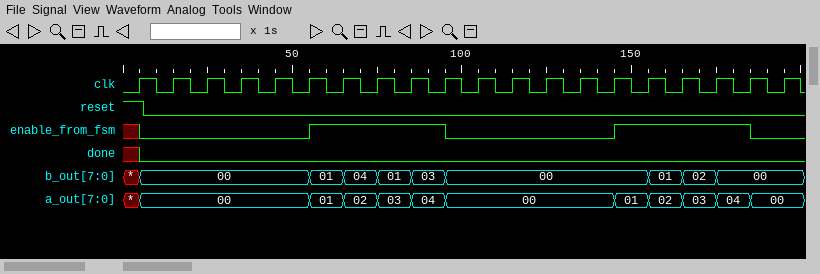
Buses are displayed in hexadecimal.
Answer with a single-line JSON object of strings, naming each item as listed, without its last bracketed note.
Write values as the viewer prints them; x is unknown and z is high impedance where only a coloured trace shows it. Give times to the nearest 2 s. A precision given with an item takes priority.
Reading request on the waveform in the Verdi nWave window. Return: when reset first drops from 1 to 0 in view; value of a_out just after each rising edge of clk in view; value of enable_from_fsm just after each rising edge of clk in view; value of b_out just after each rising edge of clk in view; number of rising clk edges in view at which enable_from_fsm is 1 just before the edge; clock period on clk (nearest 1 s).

{"when reset first drops from 1 to 0 in view": "6 s", "value of a_out just after each rising edge of clk in view": "00, 00, 00, 00, 00, 01, 02, 03, 04, 00, 00, 00, 00, 00, 01, 02, 03, 04, 00, 00", "value of enable_from_fsm just after each rising edge of clk in view": "0 0 0 0 0 1 1 1 1 0 0 0 0 0 1 1 1 1 0 0", "value of b_out just after each rising edge of clk in view": "00, 00, 00, 00, 00, 01, 04, 01, 03, 00, 00, 00, 00, 00, 00, 01, 02, 00, 00, 00", "number of rising clk edges in view at which enable_from_fsm is 1 just before the edge": "8", "clock period on clk": "10 s"}
